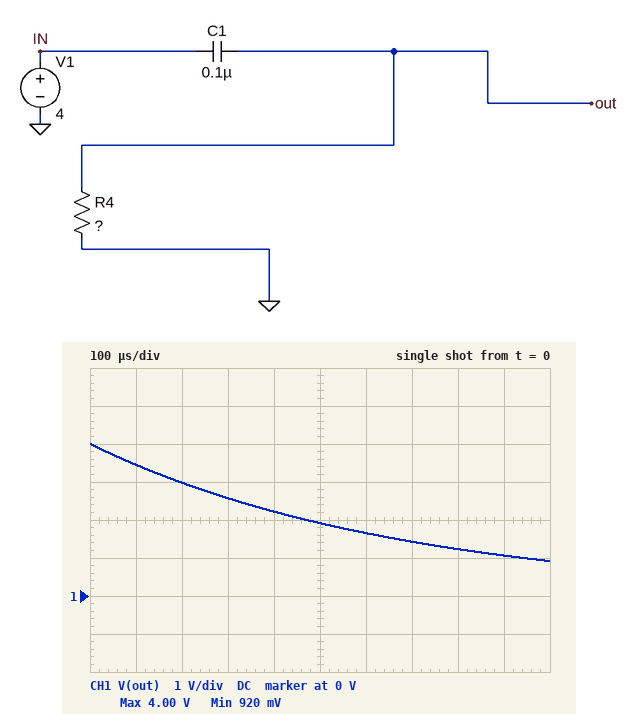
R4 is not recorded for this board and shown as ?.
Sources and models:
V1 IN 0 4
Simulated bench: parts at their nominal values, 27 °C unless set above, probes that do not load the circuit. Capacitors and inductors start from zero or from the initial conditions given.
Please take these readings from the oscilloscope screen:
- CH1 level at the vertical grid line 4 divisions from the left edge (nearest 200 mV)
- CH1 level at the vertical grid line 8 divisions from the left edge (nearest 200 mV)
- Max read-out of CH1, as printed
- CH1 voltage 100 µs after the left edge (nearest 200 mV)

2.2 V
1.2 V
4.00 V
3.4 V
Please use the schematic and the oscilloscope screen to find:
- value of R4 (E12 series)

6.8 kΩ
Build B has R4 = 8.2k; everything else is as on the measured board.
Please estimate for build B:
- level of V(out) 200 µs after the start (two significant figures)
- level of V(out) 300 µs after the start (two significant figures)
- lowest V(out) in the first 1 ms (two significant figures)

3.1 V
2.8 V
1.2 V
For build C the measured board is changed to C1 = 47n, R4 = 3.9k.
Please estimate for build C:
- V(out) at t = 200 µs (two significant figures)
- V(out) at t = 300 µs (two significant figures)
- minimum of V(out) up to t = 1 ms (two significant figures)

1.3 V
780 mV
17 mV
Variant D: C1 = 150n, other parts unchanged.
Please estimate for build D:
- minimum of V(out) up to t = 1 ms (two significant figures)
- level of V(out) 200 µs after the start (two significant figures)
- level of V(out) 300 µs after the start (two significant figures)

1.5 V
3.3 V
3.0 V
